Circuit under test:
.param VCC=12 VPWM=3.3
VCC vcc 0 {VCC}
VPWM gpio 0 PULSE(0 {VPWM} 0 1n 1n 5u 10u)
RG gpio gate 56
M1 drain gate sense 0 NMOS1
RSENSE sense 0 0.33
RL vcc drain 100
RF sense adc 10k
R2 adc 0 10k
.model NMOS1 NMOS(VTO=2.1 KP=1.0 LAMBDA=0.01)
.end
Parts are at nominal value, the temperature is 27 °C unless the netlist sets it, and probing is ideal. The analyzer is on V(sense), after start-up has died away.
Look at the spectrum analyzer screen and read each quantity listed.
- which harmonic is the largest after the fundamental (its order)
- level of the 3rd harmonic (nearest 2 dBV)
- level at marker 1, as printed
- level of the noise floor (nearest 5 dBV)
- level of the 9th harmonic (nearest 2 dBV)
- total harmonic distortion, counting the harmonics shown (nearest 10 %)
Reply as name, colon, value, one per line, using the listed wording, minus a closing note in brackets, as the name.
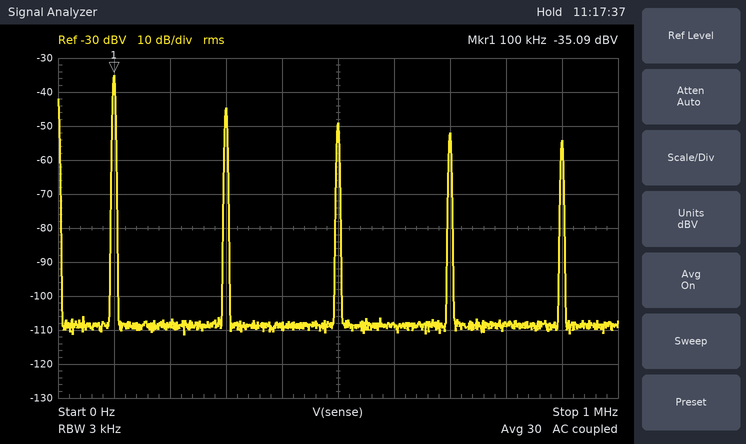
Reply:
which harmonic is the largest after the fundamental: 3
level of the 3rd harmonic: -44 dBV
level at marker 1, as printed: -35.09 dBV
level of the noise floor: -110 dBV
level of the 9th harmonic: -54 dBV
total harmonic distortion, counting the harmonics shown: 40 %
